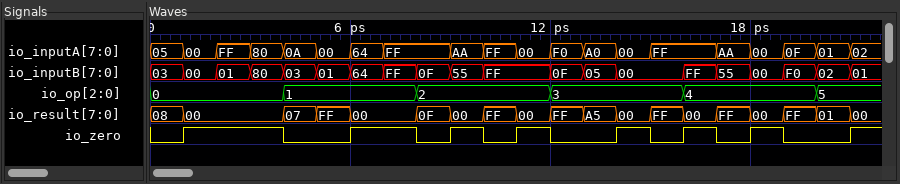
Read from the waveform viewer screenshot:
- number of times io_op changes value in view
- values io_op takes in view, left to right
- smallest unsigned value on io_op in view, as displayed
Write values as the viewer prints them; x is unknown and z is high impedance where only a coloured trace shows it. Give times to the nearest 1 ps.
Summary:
5
0, 1, 2, 3, 4, 5
0
